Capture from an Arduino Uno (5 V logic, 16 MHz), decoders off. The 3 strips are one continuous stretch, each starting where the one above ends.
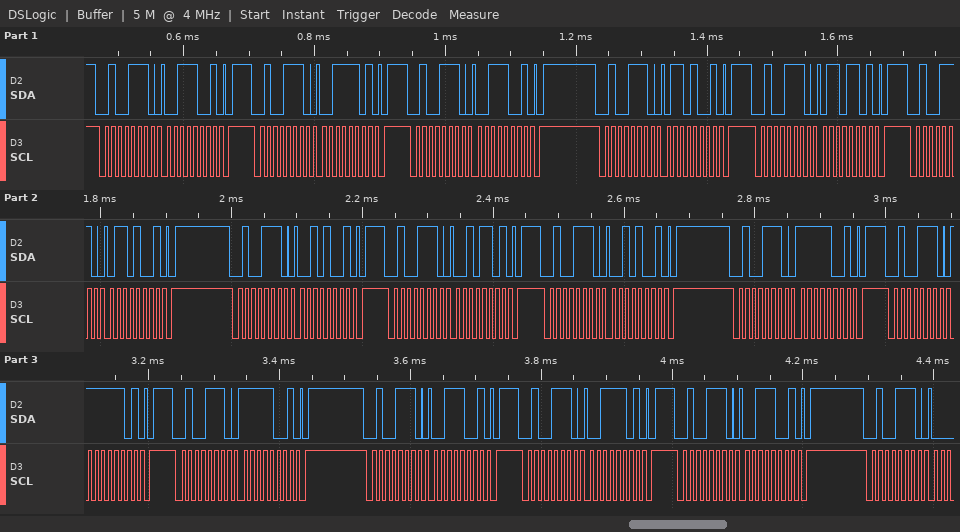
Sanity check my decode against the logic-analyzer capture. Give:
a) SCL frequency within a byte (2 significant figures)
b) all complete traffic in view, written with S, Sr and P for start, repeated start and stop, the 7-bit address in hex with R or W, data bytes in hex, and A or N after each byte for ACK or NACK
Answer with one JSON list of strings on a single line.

["100 kHz", "S 27W A 39 A P S 27W A 3D A P S 27W A 39 A P S 27W A 69 A P S 27W A 6D A P S 27W A 69 A P S 27W A 29 A P S 27W A 2D A P S 27W A 29 A P S 27W A F9 A P S 27W A FD A P S 27W A F9 A P S 27W A 39 A P S 27W A 3D A P S 27W A 39 A P S 27W A"]
